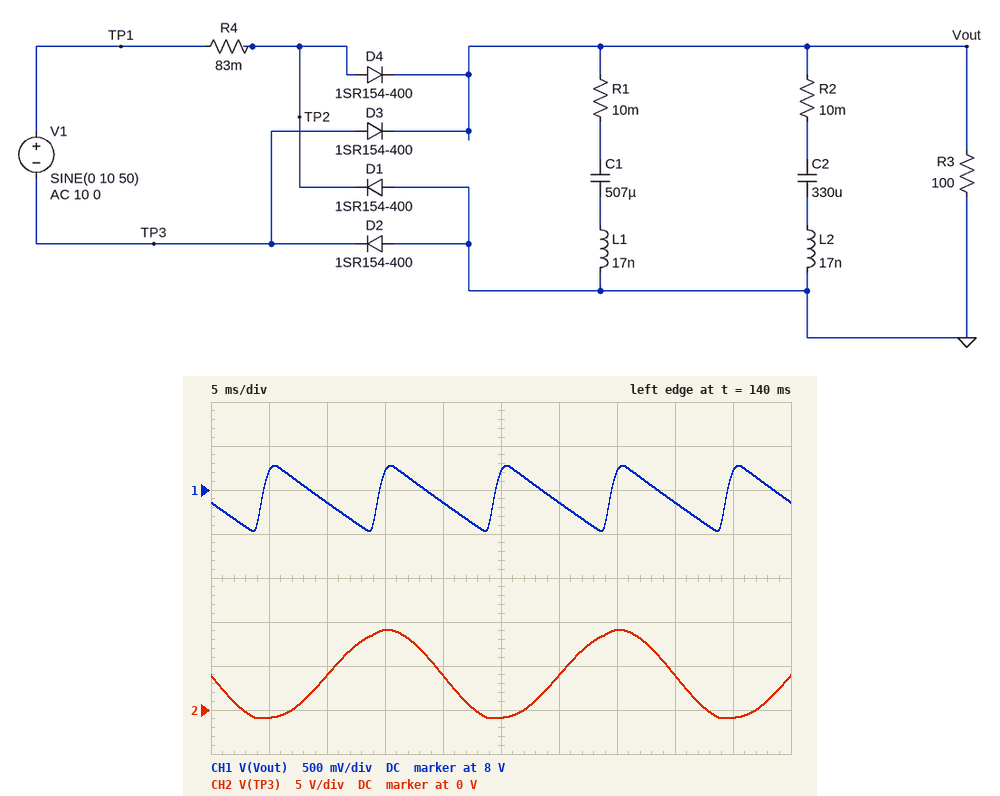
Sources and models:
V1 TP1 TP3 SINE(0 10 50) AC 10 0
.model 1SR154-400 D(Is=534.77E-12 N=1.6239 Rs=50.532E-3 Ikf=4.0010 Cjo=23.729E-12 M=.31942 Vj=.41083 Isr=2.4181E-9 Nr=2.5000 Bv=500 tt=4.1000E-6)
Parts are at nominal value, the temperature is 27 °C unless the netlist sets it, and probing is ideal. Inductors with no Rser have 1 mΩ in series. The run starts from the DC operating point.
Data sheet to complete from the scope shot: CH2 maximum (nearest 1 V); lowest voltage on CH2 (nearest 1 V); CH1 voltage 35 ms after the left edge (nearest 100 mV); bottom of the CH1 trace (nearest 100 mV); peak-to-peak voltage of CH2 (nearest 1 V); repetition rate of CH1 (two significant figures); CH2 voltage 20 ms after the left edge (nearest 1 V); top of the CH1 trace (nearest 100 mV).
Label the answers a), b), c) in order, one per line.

a) 9 V
b) -1 V
c) 8.2 V
d) 7.5 V
e) 10 V
f) 100 Hz
g) 4 V
h) 8.3 V
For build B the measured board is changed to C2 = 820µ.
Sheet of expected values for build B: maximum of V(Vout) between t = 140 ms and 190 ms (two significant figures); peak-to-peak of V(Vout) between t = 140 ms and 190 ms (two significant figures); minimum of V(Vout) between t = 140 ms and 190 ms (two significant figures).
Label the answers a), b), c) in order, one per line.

a) 8.2 V
b) 480 mV
c) 7.7 V
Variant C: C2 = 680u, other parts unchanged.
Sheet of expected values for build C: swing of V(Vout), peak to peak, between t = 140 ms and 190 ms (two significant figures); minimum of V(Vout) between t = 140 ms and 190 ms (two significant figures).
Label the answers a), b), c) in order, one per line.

a) 540 mV
b) 7.7 V
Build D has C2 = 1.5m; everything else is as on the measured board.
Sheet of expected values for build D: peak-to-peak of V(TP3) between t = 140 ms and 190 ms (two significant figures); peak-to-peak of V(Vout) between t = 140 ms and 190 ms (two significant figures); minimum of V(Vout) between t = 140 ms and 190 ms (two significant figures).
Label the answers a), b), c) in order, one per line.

a) 10 V
b) 320 mV
c) 7.9 V
